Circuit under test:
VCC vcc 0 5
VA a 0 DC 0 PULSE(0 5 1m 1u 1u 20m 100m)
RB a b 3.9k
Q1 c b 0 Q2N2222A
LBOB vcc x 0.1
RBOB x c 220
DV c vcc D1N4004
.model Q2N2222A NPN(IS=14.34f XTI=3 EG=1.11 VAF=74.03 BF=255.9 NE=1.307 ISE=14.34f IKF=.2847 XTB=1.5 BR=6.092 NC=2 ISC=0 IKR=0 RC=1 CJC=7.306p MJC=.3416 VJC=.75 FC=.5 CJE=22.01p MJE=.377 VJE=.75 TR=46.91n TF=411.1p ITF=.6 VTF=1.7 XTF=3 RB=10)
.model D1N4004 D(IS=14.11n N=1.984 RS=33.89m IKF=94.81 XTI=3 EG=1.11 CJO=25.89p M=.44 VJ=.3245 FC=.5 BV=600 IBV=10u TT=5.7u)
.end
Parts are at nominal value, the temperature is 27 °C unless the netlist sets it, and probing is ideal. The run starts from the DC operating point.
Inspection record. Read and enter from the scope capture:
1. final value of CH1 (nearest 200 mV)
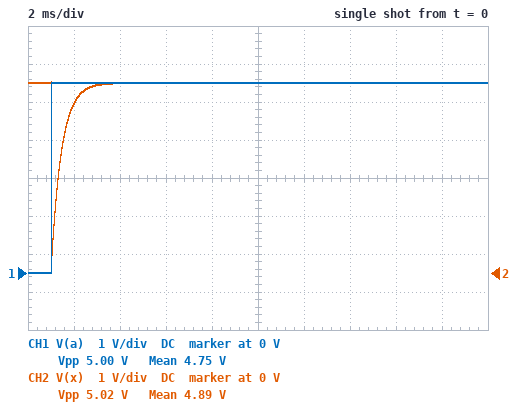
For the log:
5.0 V
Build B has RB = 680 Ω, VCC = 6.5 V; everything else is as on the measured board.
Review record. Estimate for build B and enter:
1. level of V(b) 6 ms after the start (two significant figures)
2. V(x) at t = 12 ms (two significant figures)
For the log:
820 mV
6.5 V
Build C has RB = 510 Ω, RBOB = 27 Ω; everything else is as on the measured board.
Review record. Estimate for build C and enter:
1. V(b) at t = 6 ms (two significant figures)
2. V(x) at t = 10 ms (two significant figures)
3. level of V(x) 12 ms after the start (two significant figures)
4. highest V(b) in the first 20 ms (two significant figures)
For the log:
870 mV
4.6 V
4.8 V
880 mV
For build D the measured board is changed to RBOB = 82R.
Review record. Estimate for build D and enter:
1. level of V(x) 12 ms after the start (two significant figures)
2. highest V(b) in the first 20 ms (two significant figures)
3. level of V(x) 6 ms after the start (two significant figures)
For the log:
5.0 V
770 mV
4.9 V
